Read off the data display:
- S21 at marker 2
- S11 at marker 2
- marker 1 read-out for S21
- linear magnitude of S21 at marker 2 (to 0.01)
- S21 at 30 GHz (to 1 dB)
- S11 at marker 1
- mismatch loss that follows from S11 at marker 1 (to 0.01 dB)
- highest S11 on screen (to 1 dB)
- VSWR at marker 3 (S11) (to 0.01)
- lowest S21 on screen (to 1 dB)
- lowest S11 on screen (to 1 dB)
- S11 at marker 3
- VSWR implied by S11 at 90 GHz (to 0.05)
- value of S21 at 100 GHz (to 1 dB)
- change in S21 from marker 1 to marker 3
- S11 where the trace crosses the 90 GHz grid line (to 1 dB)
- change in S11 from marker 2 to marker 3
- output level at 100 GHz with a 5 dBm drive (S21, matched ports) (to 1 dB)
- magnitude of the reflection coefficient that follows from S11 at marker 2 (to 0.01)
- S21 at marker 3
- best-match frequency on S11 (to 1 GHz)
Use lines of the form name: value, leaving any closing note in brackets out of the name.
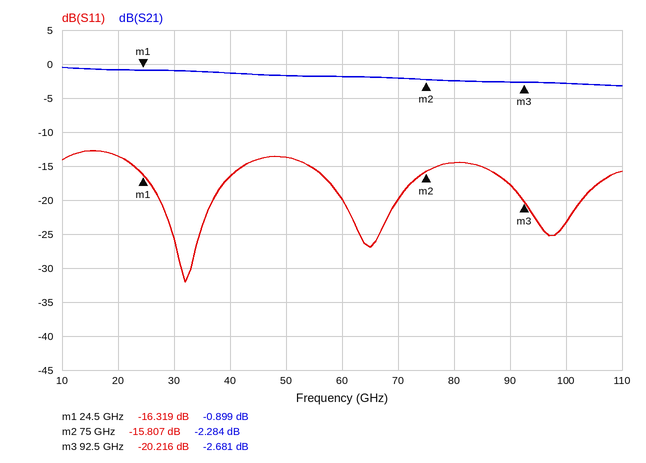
S21 at marker 2: -2.284 dB
S11 at marker 2: -15.807 dB
marker 1 read-out for S21: -0.899 dB
linear magnitude of S21 at marker 2: 0.77
S21 at 30 GHz: -1 dB
S11 at marker 1: -16.319 dB
mismatch loss that follows from S11 at marker 1: 0.10 dB
highest S11 on screen: -13 dB
VSWR at marker 3 (S11): 1.22
lowest S21 on screen: -3 dB
lowest S11 on screen: -32 dB
S11 at marker 3: -20.216 dB
VSWR implied by S11 at 90 GHz: 1.30
value of S21 at 100 GHz: -3 dB
change in S21 from marker 1 to marker 3: -1.782 dB
S11 where the trace crosses the 90 GHz grid line: -18 dB
change in S11 from marker 2 to marker 3: -4.409 dB
output level at 100 GHz with a 5 dBm drive (S21, matched ports): 2 dBm
magnitude of the reflection coefficient that follows from S11 at marker 2: 0.16
S21 at marker 3: -2.681 dB
best-match frequency on S11: 32 GHz
